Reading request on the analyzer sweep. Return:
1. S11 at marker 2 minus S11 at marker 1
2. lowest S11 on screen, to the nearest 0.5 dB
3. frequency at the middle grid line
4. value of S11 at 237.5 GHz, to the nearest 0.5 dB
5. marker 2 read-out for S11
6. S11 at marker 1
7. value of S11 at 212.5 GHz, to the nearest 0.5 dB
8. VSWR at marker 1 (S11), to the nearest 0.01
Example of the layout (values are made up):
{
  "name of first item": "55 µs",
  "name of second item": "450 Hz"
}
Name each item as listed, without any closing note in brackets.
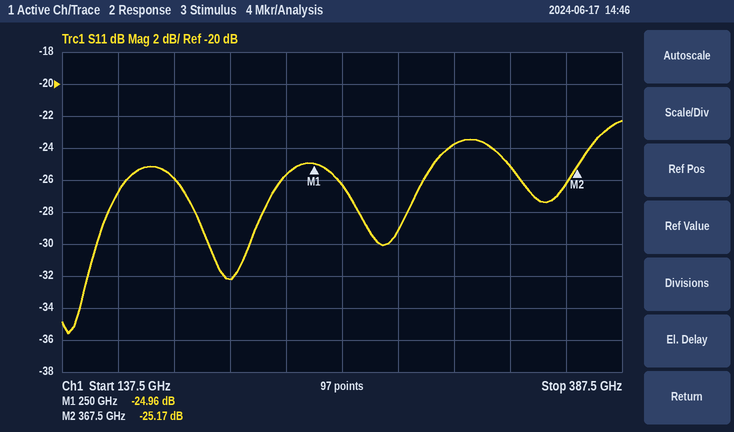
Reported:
{
  "S11 at marker 2 minus S11 at marker 1": "-0.21 dB",
  "lowest S11 on screen, to the nearest 0.5 dB": "-35.5 dB",
  "frequency at the middle grid line": "262.5 GHz",
  "value of S11 at 237.5 GHz, to the nearest 0.5 dB": "-25.5 dB",
  "marker 2 read-out for S11": "-25.17 dB",
  "S11 at marker 1": "-24.96 dB",
  "value of S11 at 212.5 GHz, to the nearest 0.5 dB": "-32.0 dB",
  "VSWR at marker 1 (S11), to the nearest 0.01": "1.12"
}
